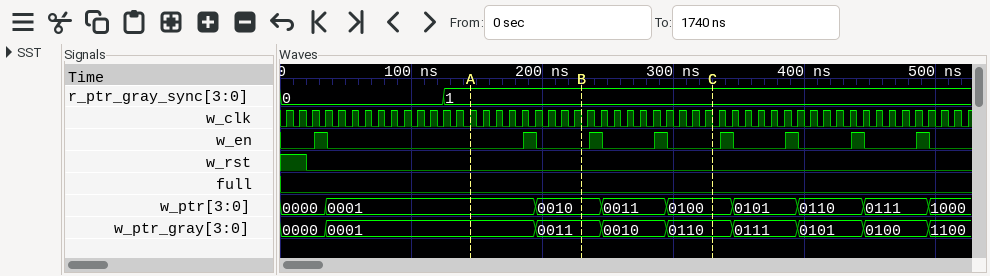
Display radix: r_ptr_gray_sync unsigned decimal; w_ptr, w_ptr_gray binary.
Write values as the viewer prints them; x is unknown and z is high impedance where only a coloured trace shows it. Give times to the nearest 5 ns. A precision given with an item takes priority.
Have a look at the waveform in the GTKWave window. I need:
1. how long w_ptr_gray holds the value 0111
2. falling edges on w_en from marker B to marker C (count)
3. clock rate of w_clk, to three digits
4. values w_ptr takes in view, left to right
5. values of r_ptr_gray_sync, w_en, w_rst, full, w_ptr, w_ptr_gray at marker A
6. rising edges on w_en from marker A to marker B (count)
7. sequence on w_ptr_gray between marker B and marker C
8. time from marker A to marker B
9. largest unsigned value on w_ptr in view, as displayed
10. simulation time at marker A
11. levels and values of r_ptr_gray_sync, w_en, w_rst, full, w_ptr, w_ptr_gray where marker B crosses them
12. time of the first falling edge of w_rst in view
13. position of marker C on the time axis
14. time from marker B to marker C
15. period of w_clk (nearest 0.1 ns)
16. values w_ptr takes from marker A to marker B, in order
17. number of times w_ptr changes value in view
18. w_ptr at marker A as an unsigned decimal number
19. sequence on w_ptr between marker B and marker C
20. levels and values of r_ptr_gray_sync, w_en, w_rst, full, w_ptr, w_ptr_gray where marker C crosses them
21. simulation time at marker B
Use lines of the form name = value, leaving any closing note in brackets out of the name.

how long w_ptr_gray holds the value 0111 = 50 ns
falling edges on w_en from marker B to marker C = 2
clock rate of w_clk, to three digits = 100 MHz
values w_ptr takes in view, left to right = 0000, 0001, 0010, 0011, 0100, 0101, 0110, 0111, 1000
values of r_ptr_gray_sync, w_en, w_rst, full, w_ptr, w_ptr_gray at marker A = r_ptr_gray_sync=1, w_en=0, w_rst=0, full=0, w_ptr=0001, w_ptr_gray=0001
rising edges on w_en from marker A to marker B = 1
sequence on w_ptr_gray between marker B and marker C = 0011, 0010, 0110
time from marker A to marker B = 85 ns
largest unsigned value on w_ptr in view, as displayed = 1000
simulation time at marker A = 145 ns
levels and values of r_ptr_gray_sync, w_en, w_rst, full, w_ptr, w_ptr_gray where marker B crosses them = r_ptr_gray_sync=1, w_en=0, w_rst=0, full=0, w_ptr=0010, w_ptr_gray=0011
time of the first falling edge of w_rst in view = 20 ns
position of marker C on the time axis = 330 ns
time from marker B to marker C = 100 ns
period of w_clk = 10 ns
values w_ptr takes from marker A to marker B, in order = 0001, 0010
number of times w_ptr changes value in view = 8
w_ptr at marker A as an unsigned decimal number = 1
sequence on w_ptr between marker B and marker C = 0010, 0011, 0100
levels and values of r_ptr_gray_sync, w_en, w_rst, full, w_ptr, w_ptr_gray where marker C crosses them = r_ptr_gray_sync=1, w_en=0, w_rst=0, full=0, w_ptr=0100, w_ptr_gray=0110
simulation time at marker B = 230 ns
